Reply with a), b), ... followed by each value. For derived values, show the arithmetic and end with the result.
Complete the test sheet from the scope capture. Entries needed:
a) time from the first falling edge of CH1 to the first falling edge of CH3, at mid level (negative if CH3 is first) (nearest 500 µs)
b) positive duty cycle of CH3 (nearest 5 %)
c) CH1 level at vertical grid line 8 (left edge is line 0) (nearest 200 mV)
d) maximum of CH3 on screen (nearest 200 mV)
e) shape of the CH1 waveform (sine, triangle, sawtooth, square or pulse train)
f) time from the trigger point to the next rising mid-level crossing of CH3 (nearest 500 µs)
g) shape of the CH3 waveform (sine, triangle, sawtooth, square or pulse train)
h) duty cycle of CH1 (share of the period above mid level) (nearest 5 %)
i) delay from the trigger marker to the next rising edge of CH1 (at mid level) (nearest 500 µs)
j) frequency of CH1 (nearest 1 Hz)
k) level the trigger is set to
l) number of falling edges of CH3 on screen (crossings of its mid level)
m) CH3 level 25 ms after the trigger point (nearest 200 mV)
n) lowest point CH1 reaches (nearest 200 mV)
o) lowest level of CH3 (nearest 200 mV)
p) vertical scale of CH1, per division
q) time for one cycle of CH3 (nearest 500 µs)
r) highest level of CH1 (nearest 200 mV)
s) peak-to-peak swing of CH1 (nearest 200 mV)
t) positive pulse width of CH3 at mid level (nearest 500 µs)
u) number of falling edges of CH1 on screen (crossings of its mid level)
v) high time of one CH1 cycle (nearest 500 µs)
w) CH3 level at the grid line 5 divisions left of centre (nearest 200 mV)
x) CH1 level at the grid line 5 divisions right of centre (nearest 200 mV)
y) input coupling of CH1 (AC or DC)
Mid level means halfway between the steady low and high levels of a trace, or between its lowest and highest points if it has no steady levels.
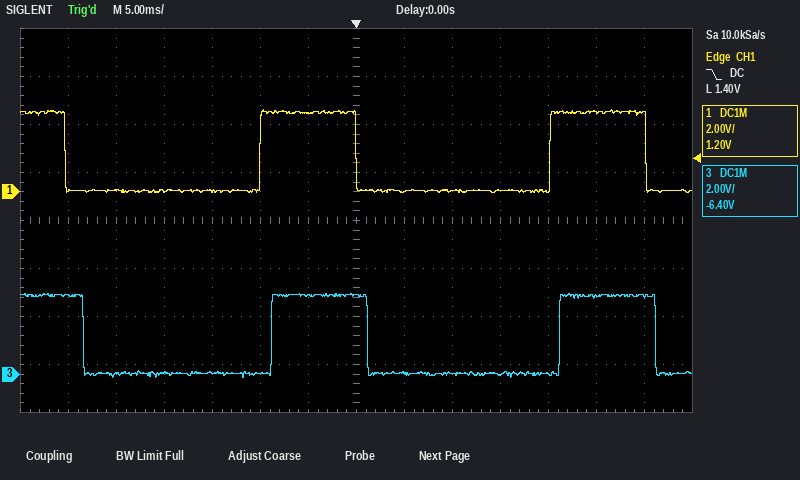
a) +2.0 ms
b) 10.0 ms / 30.0 ms ≈ 33.3 %, so 35 % to the nearest 5 %
c) 0.0 V
d) 3.4 V
e) pulse train
f) 21.0 ms
g) pulse train
h) 35 %
i) 20.0 ms
j) 33 Hz
k) 1.40 V
l) 3
m) 3.2 V
n) 0.0 V
o) -200 mV
p) 2 V
q) 30.0 ms
r) 3.4 V
s) 3.4 V − (0.0 V) = 3.4 V
t) 10.0 ms
u) 3
v) 10.0 ms
w) 0.0 V
x) 3.4 V
y) DC
